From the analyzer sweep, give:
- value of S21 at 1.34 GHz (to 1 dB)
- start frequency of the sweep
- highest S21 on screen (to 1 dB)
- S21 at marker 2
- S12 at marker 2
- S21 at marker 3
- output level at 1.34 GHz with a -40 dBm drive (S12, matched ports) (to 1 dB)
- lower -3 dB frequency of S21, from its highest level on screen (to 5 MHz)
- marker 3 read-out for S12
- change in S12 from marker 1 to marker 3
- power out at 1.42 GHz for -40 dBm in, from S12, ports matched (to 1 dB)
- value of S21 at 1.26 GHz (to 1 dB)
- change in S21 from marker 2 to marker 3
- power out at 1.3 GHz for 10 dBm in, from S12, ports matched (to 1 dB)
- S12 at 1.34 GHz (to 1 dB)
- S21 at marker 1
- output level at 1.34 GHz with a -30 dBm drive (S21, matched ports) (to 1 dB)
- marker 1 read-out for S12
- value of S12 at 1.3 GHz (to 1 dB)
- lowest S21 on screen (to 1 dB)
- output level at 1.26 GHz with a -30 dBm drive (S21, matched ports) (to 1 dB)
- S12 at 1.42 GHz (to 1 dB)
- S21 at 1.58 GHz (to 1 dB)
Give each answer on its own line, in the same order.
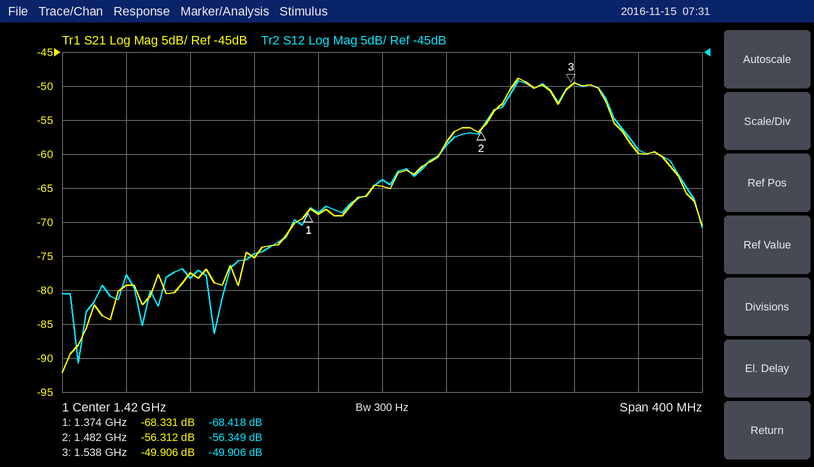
-75 dB
1.22 GHz
-49 dB
-56.312 dB
-56.349 dB
-49.906 dB
-115 dBm
1.495 GHz
-49.906 dB
18.512 dB
-104 dBm
-79 dB
6.406 dB
-68 dBm
-75 dB
-68.331 dB
-105 dBm
-68.418 dB
-78 dB
-92 dB
-109 dBm
-64 dB
-60 dB
